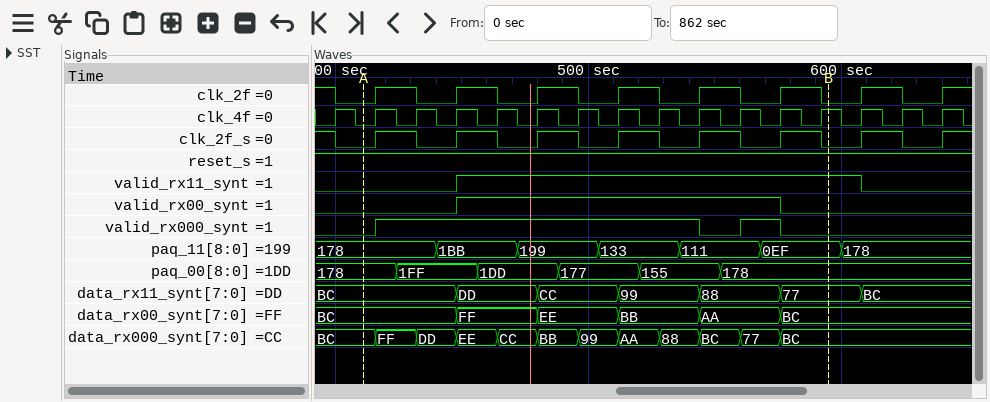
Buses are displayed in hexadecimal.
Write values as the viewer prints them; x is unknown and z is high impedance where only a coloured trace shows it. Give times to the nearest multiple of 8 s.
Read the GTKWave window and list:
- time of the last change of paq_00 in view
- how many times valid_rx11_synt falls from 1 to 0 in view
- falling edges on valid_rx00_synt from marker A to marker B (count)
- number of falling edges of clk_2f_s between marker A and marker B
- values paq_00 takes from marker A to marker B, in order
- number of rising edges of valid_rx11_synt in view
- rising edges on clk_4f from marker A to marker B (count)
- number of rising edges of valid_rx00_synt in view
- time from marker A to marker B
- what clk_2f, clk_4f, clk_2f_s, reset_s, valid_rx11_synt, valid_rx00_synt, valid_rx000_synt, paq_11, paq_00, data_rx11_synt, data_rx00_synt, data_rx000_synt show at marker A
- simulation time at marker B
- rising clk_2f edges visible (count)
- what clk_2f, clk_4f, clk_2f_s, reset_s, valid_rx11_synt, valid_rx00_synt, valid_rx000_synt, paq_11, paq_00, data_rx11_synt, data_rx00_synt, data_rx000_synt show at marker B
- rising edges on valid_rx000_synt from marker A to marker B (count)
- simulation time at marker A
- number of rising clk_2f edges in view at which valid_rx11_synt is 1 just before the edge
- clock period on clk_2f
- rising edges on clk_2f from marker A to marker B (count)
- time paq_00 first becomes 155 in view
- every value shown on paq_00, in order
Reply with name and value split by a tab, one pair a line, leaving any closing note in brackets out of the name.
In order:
time of the last change of paq_00 in view	552 s
how many times valid_rx11_synt falls from 1 to 0 in view	1
falling edges on valid_rx00_synt from marker A to marker B	1
number of falling edges of clk_2f_s between marker A and marker B	6
values paq_00 takes from marker A to marker B, in order	178, 1FF, 1DD, 177, 155, 178
number of rising edges of valid_rx11_synt in view	1
rising edges on clk_4f from marker A to marker B	12
number of rising edges of valid_rx00_synt in view	1
time from marker A to marker B	184 s
what clk_2f, clk_4f, clk_2f_s, reset_s, valid_rx11_synt, valid_rx00_synt, valid_rx000_synt, paq_11, paq_00, data_rx11_synt, data_rx00_synt, data_rx000_synt show at marker A	clk_2f=0, clk_4f=0, clk_2f_s=0, reset_s=1, valid_rx11_synt=0, valid_rx00_synt=0, valid_rx000_synt=0, paq_11=178, paq_00=178, data_rx11_synt=BC, data_rx00_synt=BC, data_rx000_synt=BC
simulation time at marker B	592 s
rising clk_2f edges visible	8
what clk_2f, clk_4f, clk_2f_s, reset_s, valid_rx11_synt, valid_rx00_synt, valid_rx000_synt, paq_11, paq_00, data_rx11_synt, data_rx00_synt, data_rx000_synt show at marker B	clk_2f=0, clk_4f=1, clk_2f_s=0, reset_s=1, valid_rx11_synt=1, valid_rx00_synt=0, valid_rx000_synt=0, paq_11=0EF, paq_00=178, data_rx11_synt=77, data_rx00_synt=BC, data_rx000_synt=BC
rising edges on valid_rx000_synt from marker A to marker B	2
simulation time at marker A	408 s
number of rising clk_2f edges in view at which valid_rx11_synt is 1 just before the edge	5
clock period on clk_2f	32 s
rising edges on clk_2f from marker A to marker B	6
time paq_00 first becomes 155 in view	520 s
every value shown on paq_00, in order	178, 1FF, 1DD, 177, 155, 178
